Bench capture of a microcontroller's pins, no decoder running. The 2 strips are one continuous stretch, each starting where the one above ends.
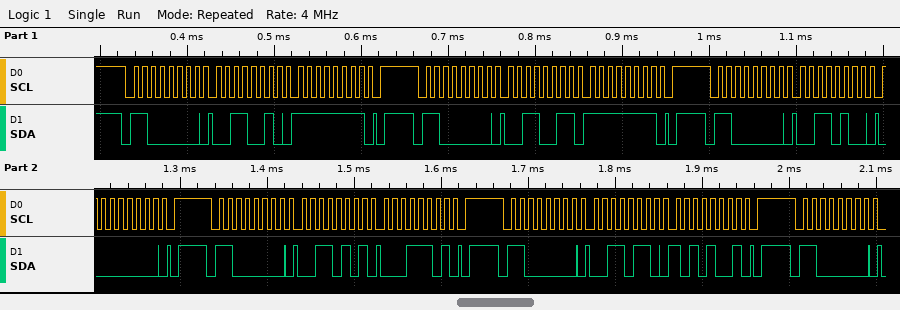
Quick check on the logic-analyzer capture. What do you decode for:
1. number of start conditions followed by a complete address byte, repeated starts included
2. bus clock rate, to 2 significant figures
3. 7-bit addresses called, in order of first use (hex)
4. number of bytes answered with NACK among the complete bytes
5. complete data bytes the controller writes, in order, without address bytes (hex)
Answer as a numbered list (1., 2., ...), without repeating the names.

1. 6
2. 100 kHz
3. 0x60
4. 0
5. 32 FF 33 FF 34 00 35 1D 36 A9
